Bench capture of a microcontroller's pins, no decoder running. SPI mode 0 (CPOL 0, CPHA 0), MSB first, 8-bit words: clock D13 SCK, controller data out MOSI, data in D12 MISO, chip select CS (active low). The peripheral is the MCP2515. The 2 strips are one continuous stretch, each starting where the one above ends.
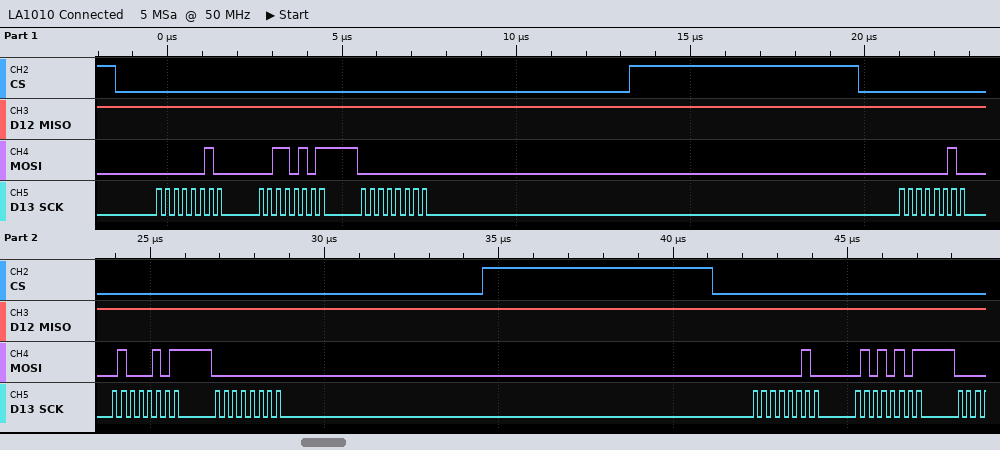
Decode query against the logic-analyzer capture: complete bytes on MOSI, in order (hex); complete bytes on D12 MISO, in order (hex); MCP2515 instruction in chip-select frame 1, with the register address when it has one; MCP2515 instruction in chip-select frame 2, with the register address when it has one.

0x02 0x35 0x00 0x02 0x45 0x00 0x02 0x55
0xFF 0xFF 0xFF 0xFF 0xFF 0xFF 0xFF 0xFF
WRITE 0x35
WRITE 0x45
